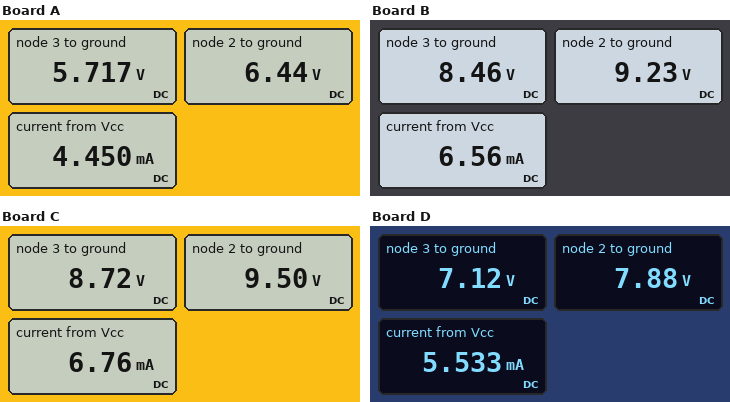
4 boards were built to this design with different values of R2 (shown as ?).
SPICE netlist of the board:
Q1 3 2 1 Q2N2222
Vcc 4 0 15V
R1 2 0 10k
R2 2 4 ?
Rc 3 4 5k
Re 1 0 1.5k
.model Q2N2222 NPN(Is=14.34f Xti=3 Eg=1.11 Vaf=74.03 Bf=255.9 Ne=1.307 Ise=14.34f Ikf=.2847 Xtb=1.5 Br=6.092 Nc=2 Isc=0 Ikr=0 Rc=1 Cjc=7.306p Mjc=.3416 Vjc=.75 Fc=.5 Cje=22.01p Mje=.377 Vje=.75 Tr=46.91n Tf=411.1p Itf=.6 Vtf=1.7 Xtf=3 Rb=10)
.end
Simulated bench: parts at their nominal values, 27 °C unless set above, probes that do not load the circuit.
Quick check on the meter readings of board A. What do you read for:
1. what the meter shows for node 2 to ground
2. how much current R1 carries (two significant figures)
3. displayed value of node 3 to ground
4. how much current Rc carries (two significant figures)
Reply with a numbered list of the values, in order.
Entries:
1. 6.44 V
2. 640 µA
3. 5.717 V
4. 1.9 mA
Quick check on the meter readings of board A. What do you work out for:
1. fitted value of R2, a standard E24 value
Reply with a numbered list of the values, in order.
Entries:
1. 3.3 kΩ
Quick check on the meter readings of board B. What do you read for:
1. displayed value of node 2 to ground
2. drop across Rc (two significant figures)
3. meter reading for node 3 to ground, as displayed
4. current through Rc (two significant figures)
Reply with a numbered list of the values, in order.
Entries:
1. 9.23 V
2. 6.5 V
3. 8.46 V
4. 1.3 mA
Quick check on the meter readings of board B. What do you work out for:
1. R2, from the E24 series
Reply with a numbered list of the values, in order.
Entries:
1. 1.1 kΩ
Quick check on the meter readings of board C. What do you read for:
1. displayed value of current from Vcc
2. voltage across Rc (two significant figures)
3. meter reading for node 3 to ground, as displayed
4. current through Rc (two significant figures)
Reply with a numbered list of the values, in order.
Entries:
1. 6.76 mA
2. 6.3 V
3. 8.72 V
4. 1.3 mA
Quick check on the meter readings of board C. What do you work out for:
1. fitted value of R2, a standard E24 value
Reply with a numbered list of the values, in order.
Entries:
1. 1 kΩ
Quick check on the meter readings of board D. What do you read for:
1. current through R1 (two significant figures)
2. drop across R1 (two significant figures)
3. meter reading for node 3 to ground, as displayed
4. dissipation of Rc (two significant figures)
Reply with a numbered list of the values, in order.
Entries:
1. 790 µA
2. 7.9 V
3. 7.12 V
4. 12 mW
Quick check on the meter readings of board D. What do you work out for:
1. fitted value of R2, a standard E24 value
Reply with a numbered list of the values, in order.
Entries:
1. 1.8 kΩ
